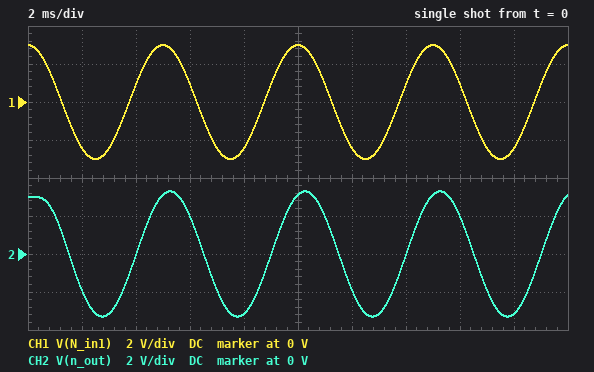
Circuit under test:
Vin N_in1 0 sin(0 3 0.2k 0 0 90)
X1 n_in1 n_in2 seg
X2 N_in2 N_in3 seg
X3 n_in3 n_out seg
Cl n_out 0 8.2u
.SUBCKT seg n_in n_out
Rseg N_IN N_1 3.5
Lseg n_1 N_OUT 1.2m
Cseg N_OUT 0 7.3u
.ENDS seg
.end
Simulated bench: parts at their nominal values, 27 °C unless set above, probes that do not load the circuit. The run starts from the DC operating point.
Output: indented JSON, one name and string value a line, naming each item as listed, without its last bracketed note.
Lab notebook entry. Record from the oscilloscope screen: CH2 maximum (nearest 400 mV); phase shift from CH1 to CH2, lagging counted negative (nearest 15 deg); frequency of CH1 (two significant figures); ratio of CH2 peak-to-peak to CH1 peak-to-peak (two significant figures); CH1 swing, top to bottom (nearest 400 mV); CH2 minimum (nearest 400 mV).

{
  "CH2 maximum": "3.2 V",
  "phase shift from CH1 to CH2, lagging counted negative": "-15 deg",
  "frequency of CH1": "200 Hz",
  "ratio of CH2 peak-to-peak to CH1 peak-to-peak": "1.1",
  "CH1 swing, top to bottom": "6.0 V",
  "CH2 minimum": "-3.2 V"
}
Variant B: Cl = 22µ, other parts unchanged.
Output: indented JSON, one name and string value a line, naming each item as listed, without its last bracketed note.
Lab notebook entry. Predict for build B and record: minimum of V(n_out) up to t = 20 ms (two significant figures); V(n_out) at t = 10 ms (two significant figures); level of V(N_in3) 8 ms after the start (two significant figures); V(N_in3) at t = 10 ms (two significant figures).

{
  "minimum of V(n_out) up to t = 20 ms": "-3.3 V",
  "V(n_out) at t = 10 ms": "2.8 V",
  "level of V(N_in3) 8 ms after the start": "-3.1 V",
  "V(N_in3) at t = 10 ms": "2.9 V"
}
